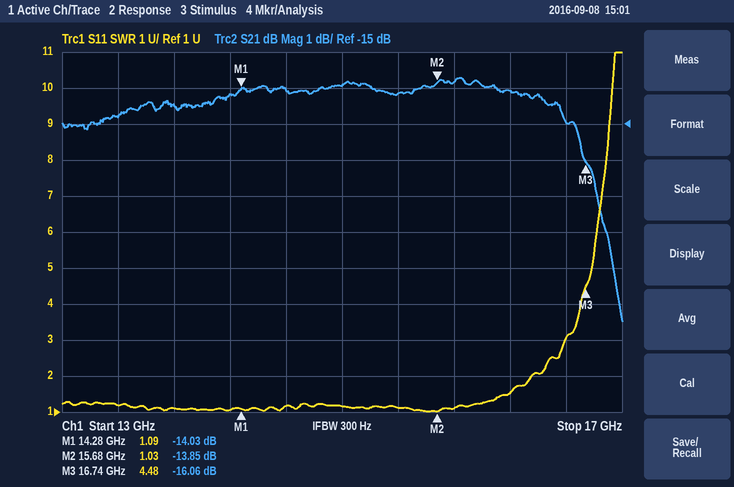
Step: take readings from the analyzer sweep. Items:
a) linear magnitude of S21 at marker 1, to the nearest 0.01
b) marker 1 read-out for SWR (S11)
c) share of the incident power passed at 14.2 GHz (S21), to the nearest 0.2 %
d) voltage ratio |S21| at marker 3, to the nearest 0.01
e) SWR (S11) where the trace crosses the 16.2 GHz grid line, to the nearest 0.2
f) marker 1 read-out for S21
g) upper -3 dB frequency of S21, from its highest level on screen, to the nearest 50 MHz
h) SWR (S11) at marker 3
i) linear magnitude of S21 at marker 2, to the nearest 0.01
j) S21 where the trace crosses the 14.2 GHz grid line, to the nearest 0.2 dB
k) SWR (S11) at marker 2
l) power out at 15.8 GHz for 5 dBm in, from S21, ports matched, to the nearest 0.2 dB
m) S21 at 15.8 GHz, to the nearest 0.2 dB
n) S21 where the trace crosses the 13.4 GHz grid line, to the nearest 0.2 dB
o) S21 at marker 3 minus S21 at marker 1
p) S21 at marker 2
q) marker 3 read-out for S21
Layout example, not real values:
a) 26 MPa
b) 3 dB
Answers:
a) 0.20
b) 1.09
c) 3.8 %
d) 0.16
e) 1.6
f) -14.03 dB
g) 16.80 GHz
h) 4.48
i) 0.20
j) -14.2 dB
k) 1.03
l) -8.8 dBm
m) -13.8 dB
n) -14.8 dB
o) -2.03 dB
p) -13.85 dB
q) -16.06 dB
